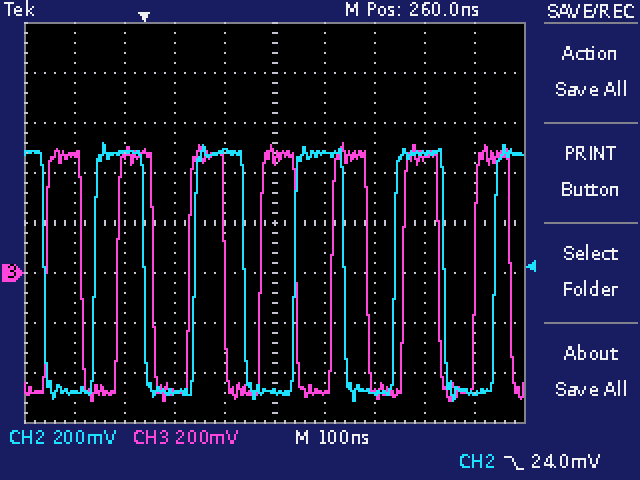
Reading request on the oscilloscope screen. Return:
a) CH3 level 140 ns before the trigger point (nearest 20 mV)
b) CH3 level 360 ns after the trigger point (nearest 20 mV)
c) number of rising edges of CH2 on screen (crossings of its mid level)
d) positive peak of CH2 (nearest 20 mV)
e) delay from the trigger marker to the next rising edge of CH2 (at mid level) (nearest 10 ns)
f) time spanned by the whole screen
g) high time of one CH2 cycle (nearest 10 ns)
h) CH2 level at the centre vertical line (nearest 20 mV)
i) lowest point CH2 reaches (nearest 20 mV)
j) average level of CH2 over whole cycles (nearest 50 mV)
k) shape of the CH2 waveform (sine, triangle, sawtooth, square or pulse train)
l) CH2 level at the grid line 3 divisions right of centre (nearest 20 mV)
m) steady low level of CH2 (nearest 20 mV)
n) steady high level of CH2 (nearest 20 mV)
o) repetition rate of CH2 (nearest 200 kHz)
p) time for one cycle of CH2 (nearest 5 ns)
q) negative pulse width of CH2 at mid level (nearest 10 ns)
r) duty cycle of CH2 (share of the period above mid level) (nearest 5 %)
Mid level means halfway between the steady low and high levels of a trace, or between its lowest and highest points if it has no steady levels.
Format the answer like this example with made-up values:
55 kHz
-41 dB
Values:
480 mV
-480 mV
5
520 mV
100 ns
1 µs
100 ns
-480 mV
-520 mV
0 mV
square
480 mV
-480 mV
480 mV
5.0 MHz
200 ns
100 ns
50 %
